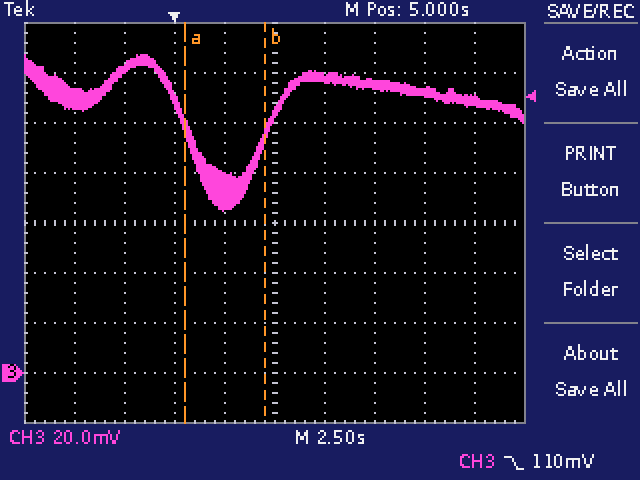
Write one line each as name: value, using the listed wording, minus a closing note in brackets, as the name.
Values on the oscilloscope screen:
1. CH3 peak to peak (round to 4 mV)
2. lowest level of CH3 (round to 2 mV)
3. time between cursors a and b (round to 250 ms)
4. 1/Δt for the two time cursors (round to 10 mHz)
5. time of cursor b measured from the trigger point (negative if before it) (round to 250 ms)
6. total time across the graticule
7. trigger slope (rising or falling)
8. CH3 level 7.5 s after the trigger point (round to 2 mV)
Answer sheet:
CH3 peak to peak: 64 mV
lowest level of CH3: 64 mV
time between cursors a and b: 4.00 s
1/Δt for the two time cursors: 250 mHz
time of cursor b measured from the trigger point (negative if before it): +4.50 s
total time across the graticule: 25 s
trigger slope: falling
CH3 level 7.5 s after the trigger point: 118 mV
